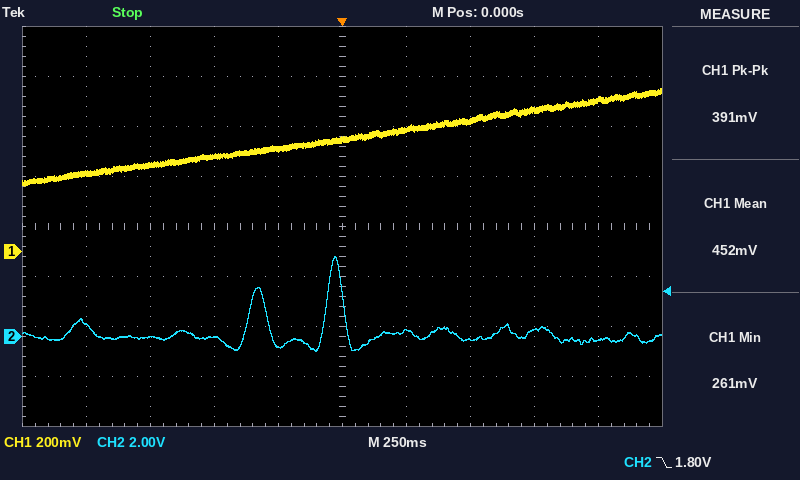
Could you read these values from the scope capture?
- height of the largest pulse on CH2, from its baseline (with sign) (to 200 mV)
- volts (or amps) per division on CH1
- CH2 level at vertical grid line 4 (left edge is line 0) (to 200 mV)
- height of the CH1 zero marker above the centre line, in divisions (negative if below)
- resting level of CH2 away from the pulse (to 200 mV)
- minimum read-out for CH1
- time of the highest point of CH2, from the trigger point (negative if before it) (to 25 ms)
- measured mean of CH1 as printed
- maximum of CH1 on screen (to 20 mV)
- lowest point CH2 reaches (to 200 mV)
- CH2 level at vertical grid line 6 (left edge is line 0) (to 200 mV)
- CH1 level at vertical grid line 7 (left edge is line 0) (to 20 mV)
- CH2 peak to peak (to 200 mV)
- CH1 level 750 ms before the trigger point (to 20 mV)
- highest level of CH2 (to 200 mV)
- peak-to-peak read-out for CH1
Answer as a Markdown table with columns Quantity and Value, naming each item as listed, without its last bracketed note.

| Quantity | Value |
|---|---|
| height of the largest pulse on CH2, from its baseline (with sign) | +3.2 V |
| volts (or amps) per division on CH1 | 200 mV |
| CH2 level at vertical grid line 4 (left edge is line 0) | -400 mV |
| height of the CH1 zero marker above the centre line, in divisions | -0.5 div |
| resting level of CH2 away from the pulse | 0.0 V |
| minimum read-out for CH1 | 261 mV |
| time of the highest point of CH2, from the trigger point (negative if before it) | -25 ms |
| measured mean of CH1 as printed | 452 mV |
| maximum of CH1 on screen | 660 mV |
| lowest point CH2 reaches | -600 mV |
| CH2 level at vertical grid line 6 (left edge is line 0) | 200 mV |
| CH1 level at vertical grid line 7 (left edge is line 0) | 520 mV |
| CH2 peak to peak | 3.8 V |
| CH1 level 750 ms before the trigger point | 340 mV |
| highest level of CH2 | 3.2 V |
| peak-to-peak read-out for CH1 | 391 mV |
